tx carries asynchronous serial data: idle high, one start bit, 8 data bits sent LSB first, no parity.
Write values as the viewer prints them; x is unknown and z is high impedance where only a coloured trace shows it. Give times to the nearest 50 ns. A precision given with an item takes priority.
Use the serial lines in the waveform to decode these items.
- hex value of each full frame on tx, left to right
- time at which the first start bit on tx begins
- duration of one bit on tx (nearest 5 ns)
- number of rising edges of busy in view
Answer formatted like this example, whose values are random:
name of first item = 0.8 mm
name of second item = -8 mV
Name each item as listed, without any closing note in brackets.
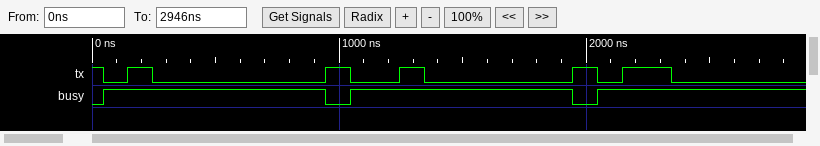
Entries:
hex value of each full frame on tx, left to right = 01, 02
time at which the first start bit on tx begins = 50 ns
duration of one bit on tx = 100 ns
number of rising edges of busy in view = 3
